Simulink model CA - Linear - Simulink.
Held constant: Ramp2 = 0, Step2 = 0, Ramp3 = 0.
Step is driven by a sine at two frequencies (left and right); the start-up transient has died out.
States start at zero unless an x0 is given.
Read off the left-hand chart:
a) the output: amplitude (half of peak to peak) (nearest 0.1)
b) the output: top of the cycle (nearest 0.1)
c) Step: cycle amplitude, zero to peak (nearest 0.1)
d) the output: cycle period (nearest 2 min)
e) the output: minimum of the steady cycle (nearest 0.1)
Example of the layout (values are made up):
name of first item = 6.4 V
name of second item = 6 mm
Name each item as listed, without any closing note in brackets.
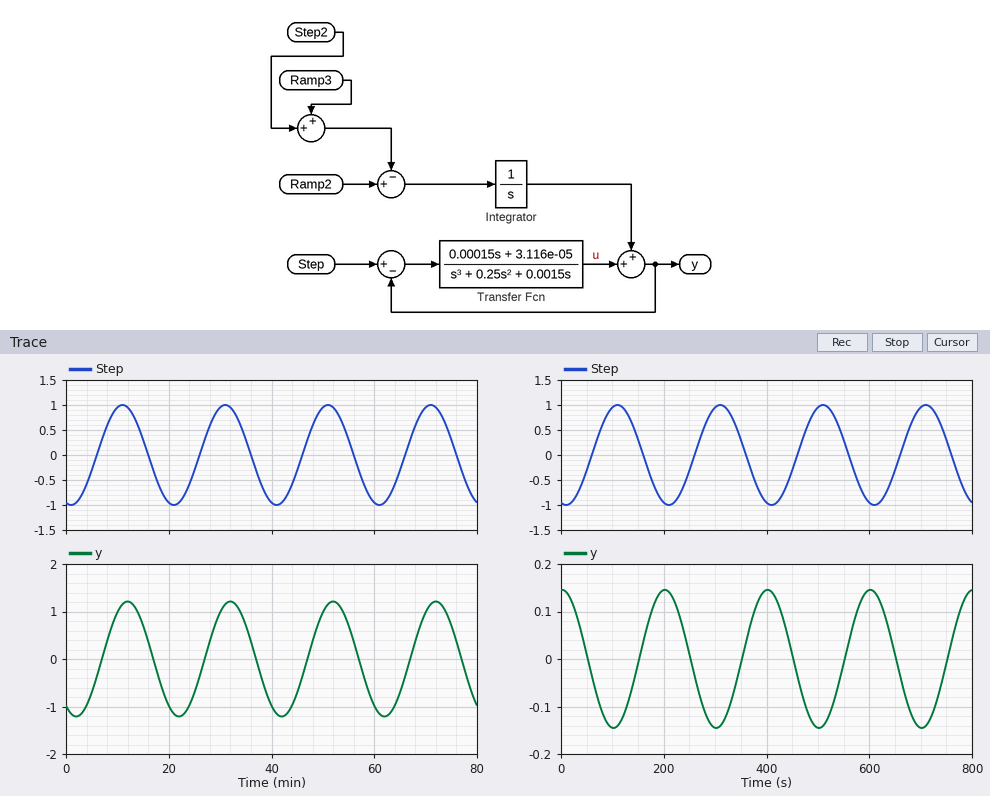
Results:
the output: amplitude (half of peak to peak) = 1.2
the output: top of the cycle = 1.2
Step: cycle amplitude, zero to peak = 1.0
the output: cycle period = 20 min
the output: minimum of the steady cycle = -1.2
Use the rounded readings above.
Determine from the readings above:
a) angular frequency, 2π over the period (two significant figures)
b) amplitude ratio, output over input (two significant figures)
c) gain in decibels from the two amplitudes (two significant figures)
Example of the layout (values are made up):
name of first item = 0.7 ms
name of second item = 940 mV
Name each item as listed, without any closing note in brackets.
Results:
angular frequency, 2π over the period = 0.31 rad/min
amplitude ratio, output over input = 1.2
gain in decibels from the two amplitudes = 1.6 dB
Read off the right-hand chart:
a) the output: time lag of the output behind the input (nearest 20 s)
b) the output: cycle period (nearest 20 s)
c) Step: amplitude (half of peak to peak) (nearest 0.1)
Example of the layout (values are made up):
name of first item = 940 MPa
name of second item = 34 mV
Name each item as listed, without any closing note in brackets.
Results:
the output: time lag of the output behind the input = 100 s
the output: cycle period = 200 s
Step: amplitude (half of peak to peak) = 1.0
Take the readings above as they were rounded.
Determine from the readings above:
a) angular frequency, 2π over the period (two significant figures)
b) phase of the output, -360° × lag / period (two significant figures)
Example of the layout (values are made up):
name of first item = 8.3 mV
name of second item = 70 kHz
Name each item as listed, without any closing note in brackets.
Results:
angular frequency, 2π over the period = 0.031 rad/s
phase of the output, -360° × lag / period = -180°
